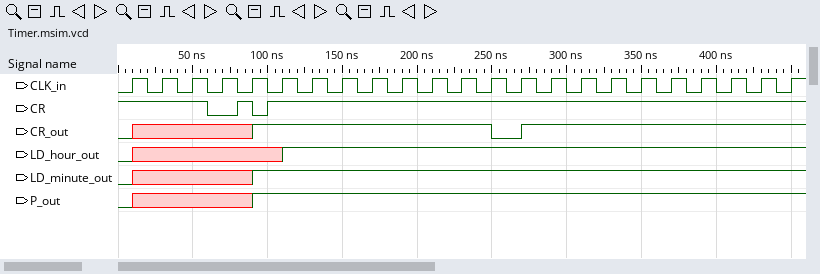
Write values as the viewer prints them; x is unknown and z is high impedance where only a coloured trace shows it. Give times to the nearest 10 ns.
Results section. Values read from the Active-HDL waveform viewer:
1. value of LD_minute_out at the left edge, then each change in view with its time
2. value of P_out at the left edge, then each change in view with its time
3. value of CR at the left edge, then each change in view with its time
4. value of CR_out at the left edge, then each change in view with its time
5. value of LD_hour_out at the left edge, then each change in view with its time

0, x at 10 ns, 1 at 90 ns
0, x at 10 ns, 1 at 90 ns
1, 0 at 60 ns, 1 at 80 ns, 0 at 90 ns, 1 at 100 ns
0, x at 10 ns, 1 at 90 ns, 0 at 250 ns, 1 at 270 ns
0, x at 10 ns, 1 at 110 ns
